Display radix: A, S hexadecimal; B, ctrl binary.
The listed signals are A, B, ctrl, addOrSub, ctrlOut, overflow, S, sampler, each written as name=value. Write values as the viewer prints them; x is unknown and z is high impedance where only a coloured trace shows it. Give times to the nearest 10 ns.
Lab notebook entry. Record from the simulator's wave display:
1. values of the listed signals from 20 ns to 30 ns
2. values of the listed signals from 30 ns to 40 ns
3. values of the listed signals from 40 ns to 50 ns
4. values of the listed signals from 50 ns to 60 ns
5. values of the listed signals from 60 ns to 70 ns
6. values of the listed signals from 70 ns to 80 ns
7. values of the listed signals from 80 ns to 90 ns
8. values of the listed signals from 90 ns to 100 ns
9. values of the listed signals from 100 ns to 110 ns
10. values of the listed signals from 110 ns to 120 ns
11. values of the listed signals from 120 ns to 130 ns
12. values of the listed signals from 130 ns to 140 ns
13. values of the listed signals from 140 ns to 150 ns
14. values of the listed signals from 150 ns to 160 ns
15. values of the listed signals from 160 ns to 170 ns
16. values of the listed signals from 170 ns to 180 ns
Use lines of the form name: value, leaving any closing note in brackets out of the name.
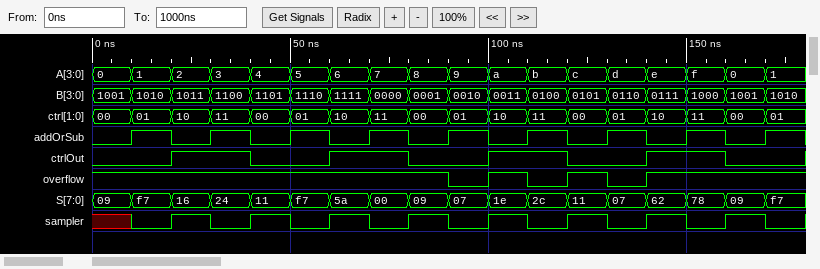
values of the listed signals from 20 ns to 30 ns: A=2, B=1011, ctrl=10, addOrSub=0, ctrlOut=1, overflow=1, S=16, sampler=1
values of the listed signals from 30 ns to 40 ns: A=3, B=1100, ctrl=11, addOrSub=1, ctrlOut=1, overflow=1, S=24, sampler=0
values of the listed signals from 40 ns to 50 ns: A=4, B=1101, ctrl=00, addOrSub=0, ctrlOut=0, overflow=1, S=11, sampler=1
values of the listed signals from 50 ns to 60 ns: A=5, B=1110, ctrl=01, addOrSub=1, ctrlOut=0, overflow=1, S=f7, sampler=0
values of the listed signals from 60 ns to 70 ns: A=6, B=1111, ctrl=10, addOrSub=0, ctrlOut=1, overflow=1, S=5a, sampler=1
values of the listed signals from 70 ns to 80 ns: A=7, B=0000, ctrl=11, addOrSub=1, ctrlOut=1, overflow=1, S=00, sampler=0
values of the listed signals from 80 ns to 90 ns: A=8, B=0001, ctrl=00, addOrSub=0, ctrlOut=0, overflow=1, S=09, sampler=1
values of the listed signals from 90 ns to 100 ns: A=9, B=0010, ctrl=01, addOrSub=1, ctrlOut=0, overflow=0, S=07, sampler=0
values of the listed signals from 100 ns to 110 ns: A=a, B=0011, ctrl=10, addOrSub=0, ctrlOut=1, overflow=1, S=1e, sampler=1
values of the listed signals from 110 ns to 120 ns: A=b, B=0100, ctrl=11, addOrSub=1, ctrlOut=1, overflow=0, S=2c, sampler=0
values of the listed signals from 120 ns to 130 ns: A=c, B=0101, ctrl=00, addOrSub=0, ctrlOut=0, overflow=1, S=11, sampler=1
values of the listed signals from 130 ns to 140 ns: A=d, B=0110, ctrl=01, addOrSub=1, ctrlOut=0, overflow=0, S=07, sampler=0
values of the listed signals from 140 ns to 150 ns: A=e, B=0111, ctrl=10, addOrSub=0, ctrlOut=1, overflow=1, S=62, sampler=1
values of the listed signals from 150 ns to 160 ns: A=f, B=1000, ctrl=11, addOrSub=1, ctrlOut=1, overflow=1, S=78, sampler=0
values of the listed signals from 160 ns to 170 ns: A=0, B=1001, ctrl=00, addOrSub=0, ctrlOut=0, overflow=1, S=09, sampler=1
values of the listed signals from 170 ns to 180 ns: A=1, B=1010, ctrl=01, addOrSub=1, ctrlOut=0, overflow=1, S=f7, sampler=0
